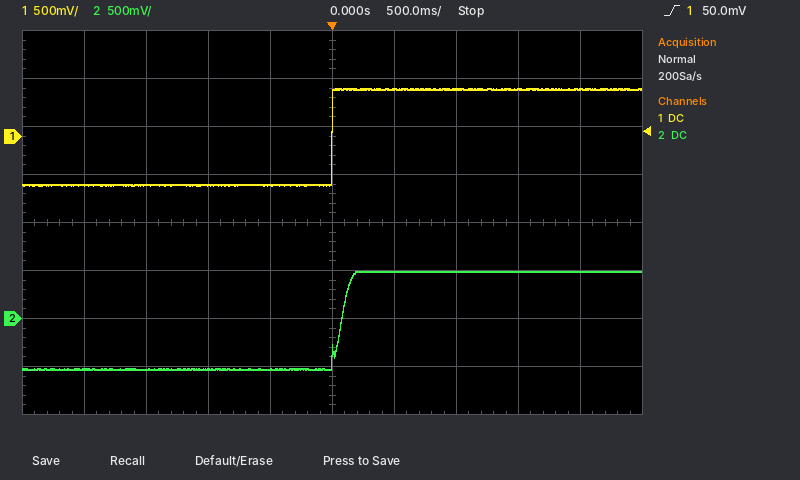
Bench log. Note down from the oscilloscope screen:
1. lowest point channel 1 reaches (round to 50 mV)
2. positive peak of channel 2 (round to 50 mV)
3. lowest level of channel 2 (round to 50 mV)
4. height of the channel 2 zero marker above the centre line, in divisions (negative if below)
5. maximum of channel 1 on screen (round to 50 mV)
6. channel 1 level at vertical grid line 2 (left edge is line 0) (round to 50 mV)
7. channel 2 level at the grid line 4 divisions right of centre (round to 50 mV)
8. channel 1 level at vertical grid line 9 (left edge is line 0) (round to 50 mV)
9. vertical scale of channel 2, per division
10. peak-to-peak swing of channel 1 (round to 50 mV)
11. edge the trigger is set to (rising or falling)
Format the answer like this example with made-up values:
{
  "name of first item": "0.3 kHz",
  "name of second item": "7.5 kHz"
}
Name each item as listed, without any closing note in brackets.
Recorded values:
{
  "lowest point channel 1 reaches": "-500 mV",
  "positive peak of channel 2": "500 mV",
  "lowest level of channel 2": "-550 mV",
  "height of the channel 2 zero marker above the centre line, in divisions": "-2.0 div",
  "maximum of channel 1 on screen": "500 mV",
  "channel 1 level at vertical grid line 2 (left edge is line 0)": "-500 mV",
  "channel 2 level at the grid line 4 divisions right of centre": "500 mV",
  "channel 1 level at vertical grid line 9 (left edge is line 0)": "500 mV",
  "vertical scale of channel 2, per division": "500 mV",
  "peak-to-peak swing of channel 1": "1.00 V",
  "edge the trigger is set to": "rising"
}
